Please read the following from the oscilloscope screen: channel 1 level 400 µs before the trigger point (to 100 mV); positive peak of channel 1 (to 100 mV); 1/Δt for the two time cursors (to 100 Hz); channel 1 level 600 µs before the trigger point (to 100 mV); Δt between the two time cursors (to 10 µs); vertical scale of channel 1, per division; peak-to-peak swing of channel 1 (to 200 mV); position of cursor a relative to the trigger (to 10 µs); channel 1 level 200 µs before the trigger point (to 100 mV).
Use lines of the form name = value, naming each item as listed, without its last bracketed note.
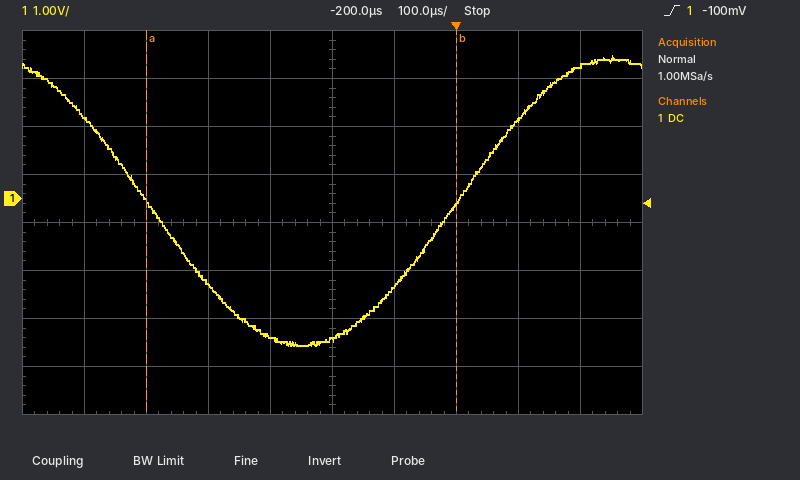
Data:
channel 1 level 400 µs before the trigger point = -1.8 V
positive peak of channel 1 = 3.0 V
1/Δt for the two time cursors = 2.0 kHz
channel 1 level 600 µs before the trigger point = 1.7 V
Δt between the two time cursors = 500 µs
vertical scale of channel 1, per division = 1 V
peak-to-peak swing of channel 1 = 6.0 V
position of cursor a relative to the trigger = -500 µs
channel 1 level 200 µs before the trigger point = -2.9 V
